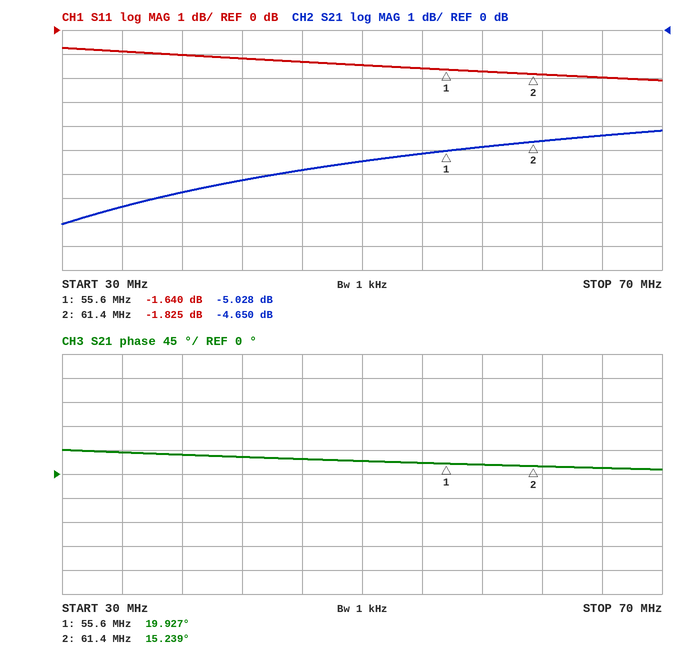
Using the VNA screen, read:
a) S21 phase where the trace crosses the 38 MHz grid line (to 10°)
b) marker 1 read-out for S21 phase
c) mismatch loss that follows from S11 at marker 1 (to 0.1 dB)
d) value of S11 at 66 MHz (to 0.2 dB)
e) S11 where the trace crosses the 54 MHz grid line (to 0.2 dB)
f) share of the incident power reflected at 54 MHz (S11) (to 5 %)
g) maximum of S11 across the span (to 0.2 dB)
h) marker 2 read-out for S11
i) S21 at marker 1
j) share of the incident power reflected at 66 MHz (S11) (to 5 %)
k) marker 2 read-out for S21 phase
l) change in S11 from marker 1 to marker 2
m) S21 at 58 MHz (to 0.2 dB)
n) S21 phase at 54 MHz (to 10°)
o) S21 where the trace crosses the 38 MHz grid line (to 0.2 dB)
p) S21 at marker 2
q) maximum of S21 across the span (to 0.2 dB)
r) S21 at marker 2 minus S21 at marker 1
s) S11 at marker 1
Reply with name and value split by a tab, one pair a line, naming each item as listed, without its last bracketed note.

S21 phase where the trace crosses the 38 MHz grid line	40°
marker 1 read-out for S21 phase	19.927°
mismatch loss that follows from S11 at marker 1	5.0 dB
value of S11 at 66 MHz	-2.0 dB
S11 where the trace crosses the 54 MHz grid line	-1.6 dB
share of the incident power reflected at 54 MHz (S11)	70 %
maximum of S11 across the span	-0.8 dB
marker 2 read-out for S11	-1.825 dB
S21 at marker 1	-5.028 dB
share of the incident power reflected at 66 MHz (S11)	65 %
marker 2 read-out for S21 phase	15.239°
change in S11 from marker 1 to marker 2	-0.185 dB
S21 at 58 MHz	-4.8 dB
S21 phase at 54 MHz	20°
S21 where the trace crosses the 38 MHz grid line	-6.8 dB
S21 at marker 2	-4.650 dB
maximum of S21 across the span	-4.2 dB
S21 at marker 2 minus S21 at marker 1	0.378 dB
S11 at marker 1	-1.640 dB
